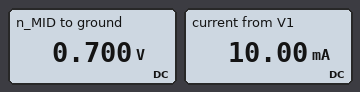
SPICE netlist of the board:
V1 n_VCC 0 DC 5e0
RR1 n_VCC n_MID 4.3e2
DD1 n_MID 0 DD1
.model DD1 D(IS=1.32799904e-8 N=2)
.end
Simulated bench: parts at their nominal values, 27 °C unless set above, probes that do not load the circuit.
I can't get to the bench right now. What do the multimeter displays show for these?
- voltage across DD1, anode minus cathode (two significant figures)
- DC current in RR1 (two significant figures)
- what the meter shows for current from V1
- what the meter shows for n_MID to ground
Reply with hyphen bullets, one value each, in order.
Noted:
- 700 mV
- 10 mA
- 10.00 mA
- 0.700 V
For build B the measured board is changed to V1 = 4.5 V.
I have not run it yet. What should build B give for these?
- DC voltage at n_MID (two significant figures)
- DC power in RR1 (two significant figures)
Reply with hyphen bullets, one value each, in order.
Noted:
- 690 mV
- 34 mW
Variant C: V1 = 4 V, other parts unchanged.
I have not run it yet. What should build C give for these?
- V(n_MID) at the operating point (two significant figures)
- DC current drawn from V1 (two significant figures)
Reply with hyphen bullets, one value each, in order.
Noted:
- 690 mV
- 7.7 mA
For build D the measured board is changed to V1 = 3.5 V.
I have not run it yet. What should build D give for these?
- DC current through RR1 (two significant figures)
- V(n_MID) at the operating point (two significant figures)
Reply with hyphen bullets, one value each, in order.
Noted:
- 6.6 mA
- 680 mV
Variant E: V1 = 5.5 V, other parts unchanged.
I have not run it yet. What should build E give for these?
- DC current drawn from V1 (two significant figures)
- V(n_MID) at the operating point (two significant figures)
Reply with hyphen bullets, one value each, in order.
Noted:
- 11 mA
- 710 mV
